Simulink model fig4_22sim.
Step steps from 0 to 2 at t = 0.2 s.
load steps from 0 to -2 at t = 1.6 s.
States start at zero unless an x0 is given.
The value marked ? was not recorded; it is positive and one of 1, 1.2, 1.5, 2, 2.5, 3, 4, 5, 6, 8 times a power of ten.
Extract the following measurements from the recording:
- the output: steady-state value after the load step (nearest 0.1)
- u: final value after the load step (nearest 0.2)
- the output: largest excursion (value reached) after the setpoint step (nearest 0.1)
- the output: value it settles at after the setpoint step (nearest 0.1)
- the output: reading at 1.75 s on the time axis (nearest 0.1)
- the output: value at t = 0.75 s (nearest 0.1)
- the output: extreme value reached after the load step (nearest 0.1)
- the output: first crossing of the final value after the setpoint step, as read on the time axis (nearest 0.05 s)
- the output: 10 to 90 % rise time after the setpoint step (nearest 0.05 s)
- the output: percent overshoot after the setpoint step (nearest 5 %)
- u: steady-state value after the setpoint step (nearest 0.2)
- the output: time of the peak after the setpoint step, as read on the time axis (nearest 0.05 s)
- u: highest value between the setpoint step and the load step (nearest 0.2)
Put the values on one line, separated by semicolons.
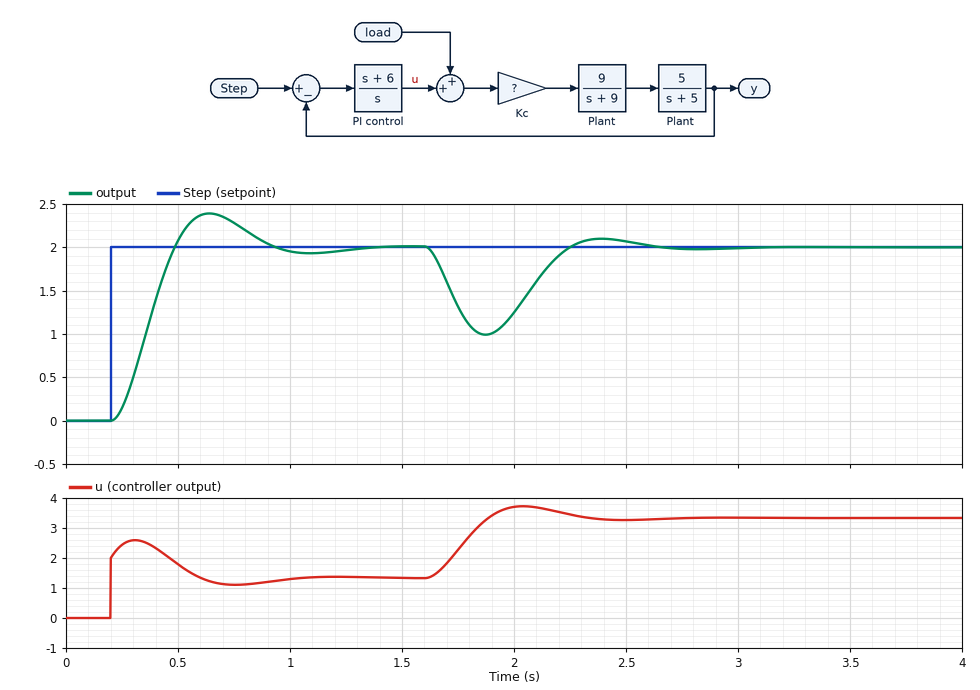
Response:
2.0; 3.4; 2.4; 2.0; 1.3; 2.3; 1.0; 0.50 s; 0.20 s; 20 %; 1.4; 0.65 s; 2.6
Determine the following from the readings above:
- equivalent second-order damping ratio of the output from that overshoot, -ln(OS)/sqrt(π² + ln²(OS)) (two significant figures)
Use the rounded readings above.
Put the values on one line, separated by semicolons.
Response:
0.46
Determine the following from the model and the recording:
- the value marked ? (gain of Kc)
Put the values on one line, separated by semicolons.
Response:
1.5
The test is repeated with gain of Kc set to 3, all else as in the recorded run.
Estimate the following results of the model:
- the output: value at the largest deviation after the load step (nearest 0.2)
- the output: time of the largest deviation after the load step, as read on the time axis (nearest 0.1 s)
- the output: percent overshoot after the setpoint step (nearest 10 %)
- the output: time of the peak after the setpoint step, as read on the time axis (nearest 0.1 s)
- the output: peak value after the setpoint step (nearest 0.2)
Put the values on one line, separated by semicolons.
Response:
0.6; 1.8 s; 30 %; 0.5 s; 2.6
